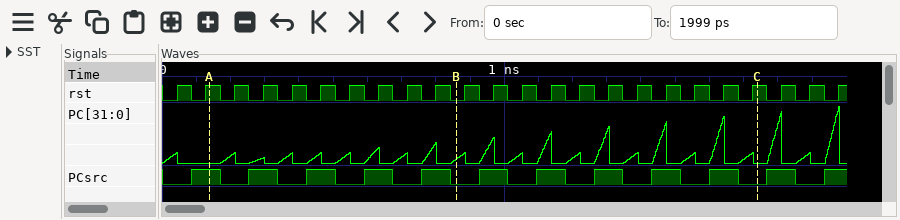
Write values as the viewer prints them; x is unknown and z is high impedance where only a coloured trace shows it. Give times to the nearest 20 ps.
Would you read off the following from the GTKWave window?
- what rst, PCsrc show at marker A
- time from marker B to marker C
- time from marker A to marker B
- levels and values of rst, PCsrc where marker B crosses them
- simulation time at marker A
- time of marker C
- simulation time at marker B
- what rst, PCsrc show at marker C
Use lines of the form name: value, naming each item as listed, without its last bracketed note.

what rst, PCsrc show at marker A: rst=1, PCsrc=1
time from marker B to marker C: 880 ps
time from marker A to marker B: 720 ps
levels and values of rst, PCsrc where marker B crosses them: rst=0, PCsrc=0
simulation time at marker A: 140 ps
time of marker C: 1740 ps
simulation time at marker B: 860 ps
what rst, PCsrc show at marker C: rst=1, PCsrc=0
